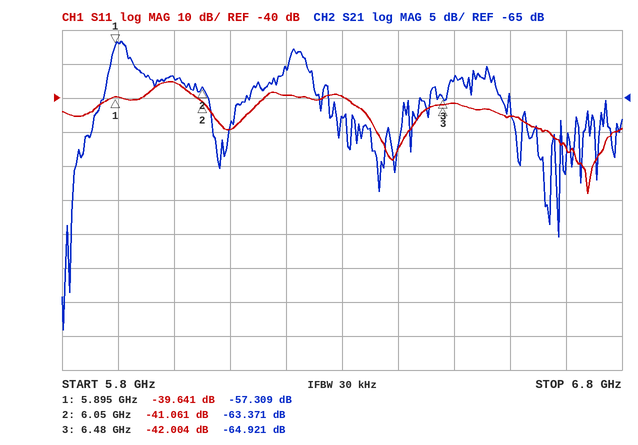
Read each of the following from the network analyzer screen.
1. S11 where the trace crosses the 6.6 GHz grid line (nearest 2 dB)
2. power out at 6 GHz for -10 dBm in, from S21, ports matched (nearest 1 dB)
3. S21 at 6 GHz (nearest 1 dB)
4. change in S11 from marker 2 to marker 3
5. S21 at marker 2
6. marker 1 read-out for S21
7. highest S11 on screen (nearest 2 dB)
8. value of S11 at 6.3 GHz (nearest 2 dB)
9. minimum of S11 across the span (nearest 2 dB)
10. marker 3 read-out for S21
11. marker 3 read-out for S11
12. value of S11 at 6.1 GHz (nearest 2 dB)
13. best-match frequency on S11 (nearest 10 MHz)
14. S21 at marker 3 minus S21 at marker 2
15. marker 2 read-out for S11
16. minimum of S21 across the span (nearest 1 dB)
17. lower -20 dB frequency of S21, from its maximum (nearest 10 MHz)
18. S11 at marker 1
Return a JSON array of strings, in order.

["-46 dB", "-72 dBm", "-62 dB", "-0.943 dB", "-63.371 dB", "-57.309 dB", "-36 dB", "-40 dB", "-68 dB", "-64.921 dB", "-42.004 dB", "-50 dB", "6.74 GHz", "-1.550 dB", "-41.061 dB", "-99 dB", "5.82 GHz", "-39.641 dB"]
